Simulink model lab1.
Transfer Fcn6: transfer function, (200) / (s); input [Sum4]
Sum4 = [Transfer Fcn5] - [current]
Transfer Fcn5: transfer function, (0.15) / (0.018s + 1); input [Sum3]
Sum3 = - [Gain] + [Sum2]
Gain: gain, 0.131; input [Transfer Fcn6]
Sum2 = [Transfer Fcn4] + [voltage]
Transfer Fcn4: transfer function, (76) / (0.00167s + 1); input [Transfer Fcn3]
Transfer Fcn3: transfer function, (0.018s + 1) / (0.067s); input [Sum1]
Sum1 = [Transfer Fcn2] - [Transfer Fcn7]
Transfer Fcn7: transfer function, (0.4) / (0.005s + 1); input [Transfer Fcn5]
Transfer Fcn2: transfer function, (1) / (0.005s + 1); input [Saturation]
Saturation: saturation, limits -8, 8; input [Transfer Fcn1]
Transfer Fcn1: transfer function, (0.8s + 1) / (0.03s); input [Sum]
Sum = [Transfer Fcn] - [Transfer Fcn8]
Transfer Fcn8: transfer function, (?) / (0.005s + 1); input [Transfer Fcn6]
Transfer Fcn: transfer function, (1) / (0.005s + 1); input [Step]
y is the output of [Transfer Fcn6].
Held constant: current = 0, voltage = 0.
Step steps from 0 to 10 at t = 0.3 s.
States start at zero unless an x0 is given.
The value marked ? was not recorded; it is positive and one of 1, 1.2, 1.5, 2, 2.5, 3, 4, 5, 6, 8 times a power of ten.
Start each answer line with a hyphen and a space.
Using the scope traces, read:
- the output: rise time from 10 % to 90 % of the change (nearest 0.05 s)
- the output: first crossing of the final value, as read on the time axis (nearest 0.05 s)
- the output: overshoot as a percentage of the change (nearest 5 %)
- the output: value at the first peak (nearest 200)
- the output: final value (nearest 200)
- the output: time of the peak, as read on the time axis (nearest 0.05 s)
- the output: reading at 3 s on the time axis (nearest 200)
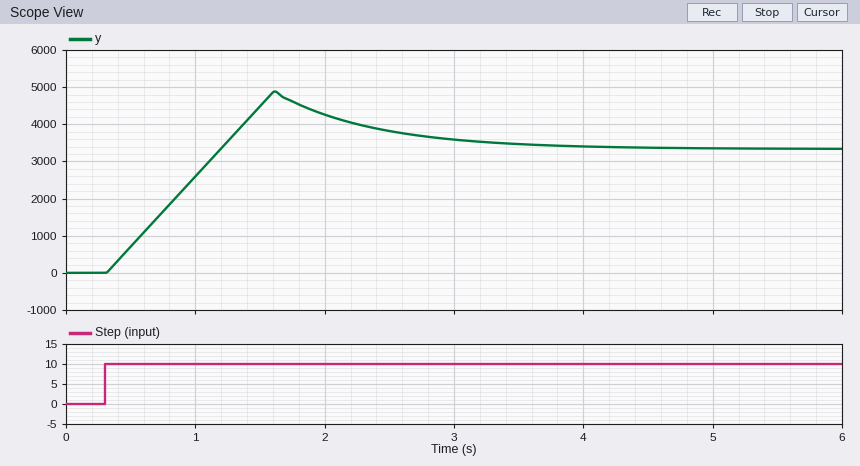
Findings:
- 0.70 s
- 1.20 s
- 45 %
- 4800
- 3400
- 1.60 s
- 3600
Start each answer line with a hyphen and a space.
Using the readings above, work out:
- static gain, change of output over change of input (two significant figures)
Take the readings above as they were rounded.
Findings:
- 340
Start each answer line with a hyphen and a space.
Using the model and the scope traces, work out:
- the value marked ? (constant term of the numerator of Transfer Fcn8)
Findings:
- 0.003
